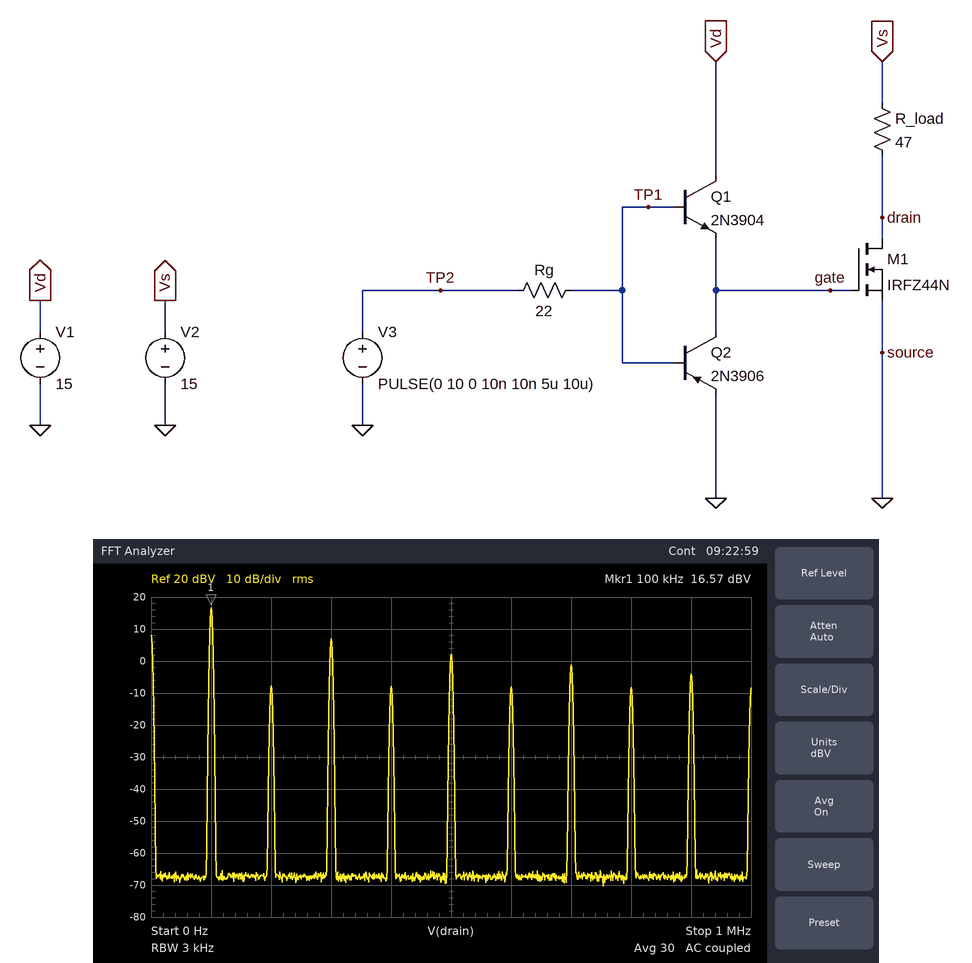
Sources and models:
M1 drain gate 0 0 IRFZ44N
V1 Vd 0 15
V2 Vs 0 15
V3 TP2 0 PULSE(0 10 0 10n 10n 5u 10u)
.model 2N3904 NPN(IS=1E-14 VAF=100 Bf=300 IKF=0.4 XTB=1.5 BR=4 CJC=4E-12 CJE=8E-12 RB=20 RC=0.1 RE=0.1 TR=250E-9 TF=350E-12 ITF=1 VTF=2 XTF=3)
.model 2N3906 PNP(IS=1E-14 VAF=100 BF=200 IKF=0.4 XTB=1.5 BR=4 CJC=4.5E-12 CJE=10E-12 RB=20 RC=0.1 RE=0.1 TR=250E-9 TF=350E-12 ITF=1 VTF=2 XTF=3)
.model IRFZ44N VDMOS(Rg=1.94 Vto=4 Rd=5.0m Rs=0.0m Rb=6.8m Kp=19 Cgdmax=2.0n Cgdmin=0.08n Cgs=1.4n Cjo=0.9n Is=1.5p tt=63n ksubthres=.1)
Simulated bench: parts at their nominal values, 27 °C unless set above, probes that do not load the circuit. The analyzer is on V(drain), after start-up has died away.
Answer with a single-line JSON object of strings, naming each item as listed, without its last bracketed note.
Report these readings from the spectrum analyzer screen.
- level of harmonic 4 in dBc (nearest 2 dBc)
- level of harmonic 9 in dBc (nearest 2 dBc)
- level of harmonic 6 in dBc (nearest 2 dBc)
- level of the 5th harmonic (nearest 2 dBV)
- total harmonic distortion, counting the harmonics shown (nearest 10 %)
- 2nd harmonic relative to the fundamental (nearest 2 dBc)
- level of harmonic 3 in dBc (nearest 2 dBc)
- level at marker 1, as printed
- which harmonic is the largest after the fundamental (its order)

{"level of harmonic 4 in dBc": "-24 dBc", "level of harmonic 9 in dBc": "-20 dBc", "level of harmonic 6 in dBc": "-24 dBc", "level of the 5th harmonic": "2 dBV", "total harmonic distortion, counting the harmonics shown": "40 %", "2nd harmonic relative to the fundamental": "-24 dBc", "level of harmonic 3 in dBc": "-10 dBc", "level at marker 1, as printed": "16.57 dBV", "which harmonic is the largest after the fundamental": "3"}
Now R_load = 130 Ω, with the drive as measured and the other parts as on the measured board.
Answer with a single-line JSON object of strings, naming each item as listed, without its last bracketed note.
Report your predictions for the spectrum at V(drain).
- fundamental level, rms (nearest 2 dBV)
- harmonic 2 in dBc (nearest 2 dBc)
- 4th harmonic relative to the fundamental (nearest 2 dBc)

{"fundamental level, rms": "16 dBV", "harmonic 2 in dBc": "-22 dBc", "4th harmonic relative to the fundamental": "-22 dBc"}
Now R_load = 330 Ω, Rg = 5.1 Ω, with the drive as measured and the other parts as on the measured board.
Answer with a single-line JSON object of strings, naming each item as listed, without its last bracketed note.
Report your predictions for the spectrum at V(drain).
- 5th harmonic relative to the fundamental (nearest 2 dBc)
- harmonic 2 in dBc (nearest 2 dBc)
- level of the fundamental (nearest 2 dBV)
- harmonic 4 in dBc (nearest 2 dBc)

{"5th harmonic relative to the fundamental": "-16 dBc", "harmonic 2 in dBc": "-18 dBc", "level of the fundamental": "16 dBV", "harmonic 4 in dBc": "-18 dBc"}
